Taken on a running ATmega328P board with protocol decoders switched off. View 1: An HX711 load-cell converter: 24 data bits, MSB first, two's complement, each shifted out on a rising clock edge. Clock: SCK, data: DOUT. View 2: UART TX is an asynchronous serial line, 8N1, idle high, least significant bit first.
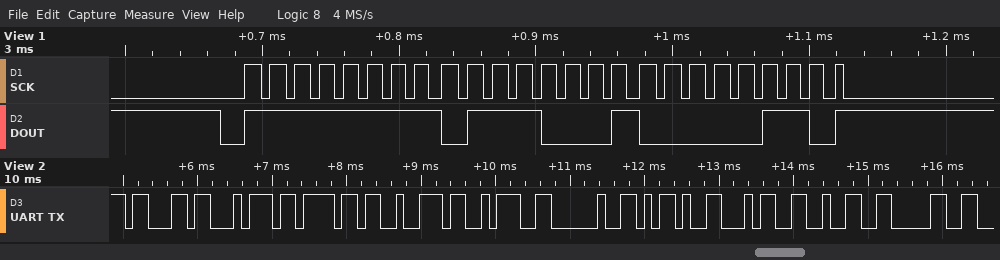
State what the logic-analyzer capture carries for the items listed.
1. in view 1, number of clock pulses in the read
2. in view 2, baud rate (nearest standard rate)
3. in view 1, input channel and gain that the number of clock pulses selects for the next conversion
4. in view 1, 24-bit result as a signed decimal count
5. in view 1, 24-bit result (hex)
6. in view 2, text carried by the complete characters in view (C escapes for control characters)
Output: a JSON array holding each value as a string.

["25", "9600 baud", "channel A, gain 128", "-36602", "0xFF7106", "\"ctor: -420\""]
